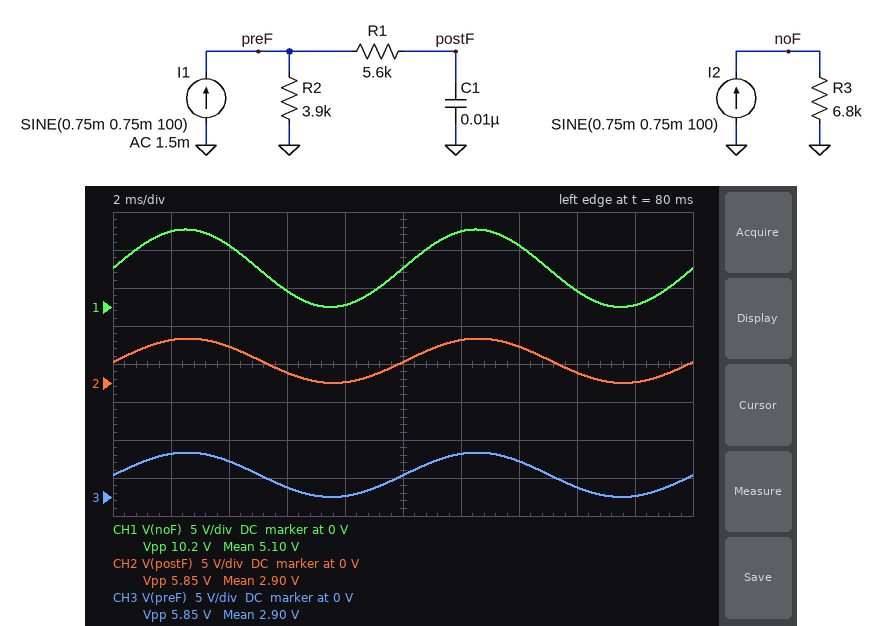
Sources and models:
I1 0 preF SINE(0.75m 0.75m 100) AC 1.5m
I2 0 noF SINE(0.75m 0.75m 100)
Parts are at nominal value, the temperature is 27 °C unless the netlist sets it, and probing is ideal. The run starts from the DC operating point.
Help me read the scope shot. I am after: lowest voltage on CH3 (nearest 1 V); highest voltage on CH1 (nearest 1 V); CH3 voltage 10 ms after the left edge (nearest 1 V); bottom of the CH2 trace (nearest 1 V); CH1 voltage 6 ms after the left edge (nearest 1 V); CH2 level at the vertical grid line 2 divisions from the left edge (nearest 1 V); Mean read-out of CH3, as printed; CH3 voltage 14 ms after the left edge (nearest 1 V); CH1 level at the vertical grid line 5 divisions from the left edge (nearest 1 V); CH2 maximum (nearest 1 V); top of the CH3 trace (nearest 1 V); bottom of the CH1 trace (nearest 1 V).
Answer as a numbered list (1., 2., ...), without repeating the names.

1. 0 V
2. 10 V
3. 3 V
4. 0 V
5. 2 V
6. 5 V
7. 2.90 V
8. 5 V
9. 5 V
10. 6 V
11. 6 V
12. 0 V
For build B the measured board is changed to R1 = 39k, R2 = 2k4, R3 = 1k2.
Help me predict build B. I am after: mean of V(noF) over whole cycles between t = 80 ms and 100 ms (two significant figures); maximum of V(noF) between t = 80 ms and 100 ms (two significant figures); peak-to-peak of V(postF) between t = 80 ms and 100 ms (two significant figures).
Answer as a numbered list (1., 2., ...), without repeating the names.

1. 900 mV
2. 1.8 V
3. 3.5 V
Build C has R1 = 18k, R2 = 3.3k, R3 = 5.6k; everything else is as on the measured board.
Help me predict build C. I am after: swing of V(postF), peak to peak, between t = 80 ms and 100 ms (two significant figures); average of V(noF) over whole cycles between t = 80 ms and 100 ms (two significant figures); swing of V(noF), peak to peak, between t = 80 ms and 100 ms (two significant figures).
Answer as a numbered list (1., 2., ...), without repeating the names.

1. 4.9 V
2. 4.2 V
3. 8.4 V
